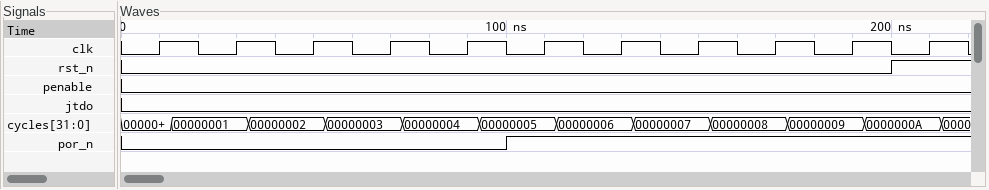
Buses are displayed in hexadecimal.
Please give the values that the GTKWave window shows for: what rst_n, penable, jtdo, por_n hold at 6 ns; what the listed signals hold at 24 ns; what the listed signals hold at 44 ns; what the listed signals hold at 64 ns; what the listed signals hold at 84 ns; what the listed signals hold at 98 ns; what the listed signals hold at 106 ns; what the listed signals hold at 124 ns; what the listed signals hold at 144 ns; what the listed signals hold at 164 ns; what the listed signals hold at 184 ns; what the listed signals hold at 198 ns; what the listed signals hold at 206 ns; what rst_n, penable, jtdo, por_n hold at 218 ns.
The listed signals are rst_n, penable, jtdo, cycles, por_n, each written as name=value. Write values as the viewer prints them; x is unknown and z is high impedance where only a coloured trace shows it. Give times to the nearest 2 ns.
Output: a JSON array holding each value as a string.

["rst_n=0, penable=0, jtdo=0, por_n=0", "rst_n=0, penable=0, jtdo=0, cycles=00000001, por_n=0", "rst_n=0, penable=0, jtdo=0, cycles=00000002, por_n=0", "rst_n=0, penable=0, jtdo=0, cycles=00000003, por_n=0", "rst_n=0, penable=0, jtdo=0, cycles=00000004, por_n=0", "rst_n=0, penable=0, jtdo=0, cycles=00000005, por_n=0", "rst_n=0, penable=0, jtdo=0, cycles=00000005, por_n=1", "rst_n=0, penable=0, jtdo=0, cycles=00000006, por_n=1", "rst_n=0, penable=0, jtdo=0, cycles=00000007, por_n=1", "rst_n=0, penable=0, jtdo=0, cycles=00000008, por_n=1", "rst_n=0, penable=0, jtdo=0, cycles=00000009, por_n=1", "rst_n=0, penable=0, jtdo=0, cycles=0000000A, por_n=1", "rst_n=1, penable=0, jtdo=0, cycles=0000000A, por_n=1", "rst_n=1, penable=0, jtdo=0, por_n=1"]
